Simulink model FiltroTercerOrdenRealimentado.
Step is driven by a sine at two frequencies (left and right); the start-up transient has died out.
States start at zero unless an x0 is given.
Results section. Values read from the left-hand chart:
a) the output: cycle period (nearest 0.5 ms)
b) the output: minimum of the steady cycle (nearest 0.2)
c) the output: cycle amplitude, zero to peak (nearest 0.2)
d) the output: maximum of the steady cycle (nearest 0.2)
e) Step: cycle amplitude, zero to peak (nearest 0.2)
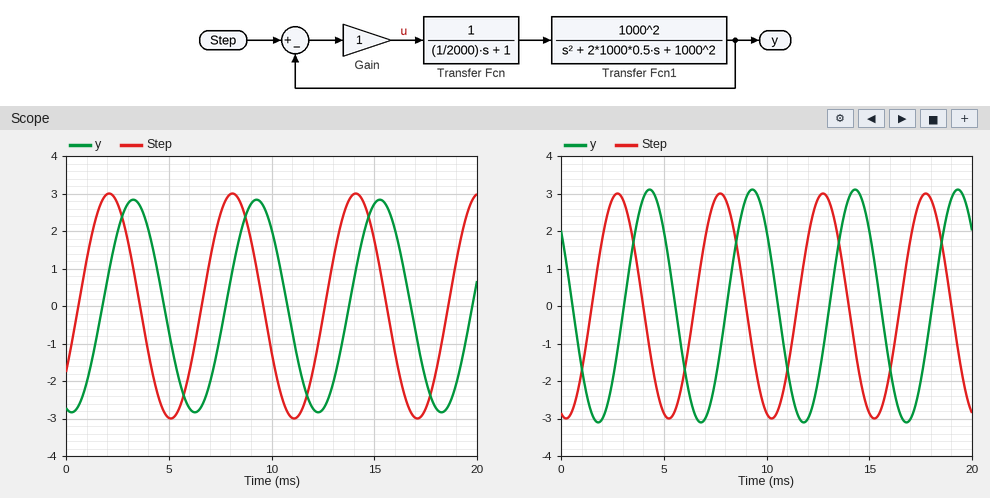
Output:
6.0 ms
-2.8
2.8
2.8
3.0
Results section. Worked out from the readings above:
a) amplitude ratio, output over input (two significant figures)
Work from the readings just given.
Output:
0.93
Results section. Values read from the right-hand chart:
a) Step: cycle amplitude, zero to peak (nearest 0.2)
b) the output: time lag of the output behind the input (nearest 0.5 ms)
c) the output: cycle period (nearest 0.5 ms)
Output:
3.0
1.5 ms
5.0 ms
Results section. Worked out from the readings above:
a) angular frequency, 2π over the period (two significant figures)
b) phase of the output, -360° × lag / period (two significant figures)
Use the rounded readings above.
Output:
1.3 rad/ms
-110°
